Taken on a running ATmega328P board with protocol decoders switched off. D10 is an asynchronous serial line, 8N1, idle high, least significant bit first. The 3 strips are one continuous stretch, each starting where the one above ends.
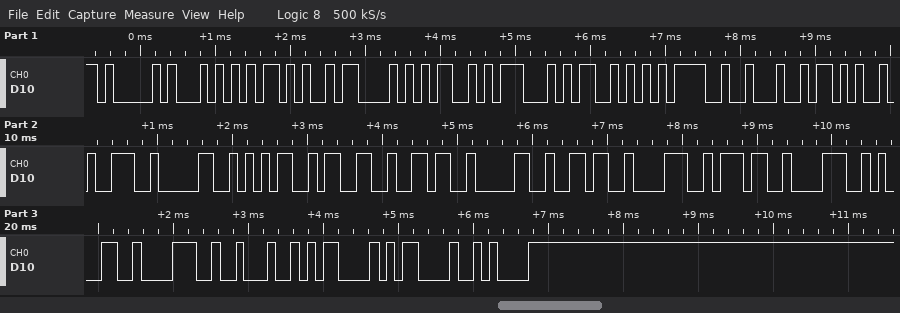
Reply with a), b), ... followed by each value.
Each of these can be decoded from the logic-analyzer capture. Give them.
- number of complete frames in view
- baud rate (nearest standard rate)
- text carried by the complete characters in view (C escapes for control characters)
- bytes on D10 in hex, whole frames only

a) 26
b) 9600 baud
c) "AT+CMGS=\"+905360687818\"\r\r\n"
d) 41 54 2B 43 4D 47 53 3D 22 2B 39 30 35 33 36 30 36 38 37 38 31 38 22 0D 0D 0A
